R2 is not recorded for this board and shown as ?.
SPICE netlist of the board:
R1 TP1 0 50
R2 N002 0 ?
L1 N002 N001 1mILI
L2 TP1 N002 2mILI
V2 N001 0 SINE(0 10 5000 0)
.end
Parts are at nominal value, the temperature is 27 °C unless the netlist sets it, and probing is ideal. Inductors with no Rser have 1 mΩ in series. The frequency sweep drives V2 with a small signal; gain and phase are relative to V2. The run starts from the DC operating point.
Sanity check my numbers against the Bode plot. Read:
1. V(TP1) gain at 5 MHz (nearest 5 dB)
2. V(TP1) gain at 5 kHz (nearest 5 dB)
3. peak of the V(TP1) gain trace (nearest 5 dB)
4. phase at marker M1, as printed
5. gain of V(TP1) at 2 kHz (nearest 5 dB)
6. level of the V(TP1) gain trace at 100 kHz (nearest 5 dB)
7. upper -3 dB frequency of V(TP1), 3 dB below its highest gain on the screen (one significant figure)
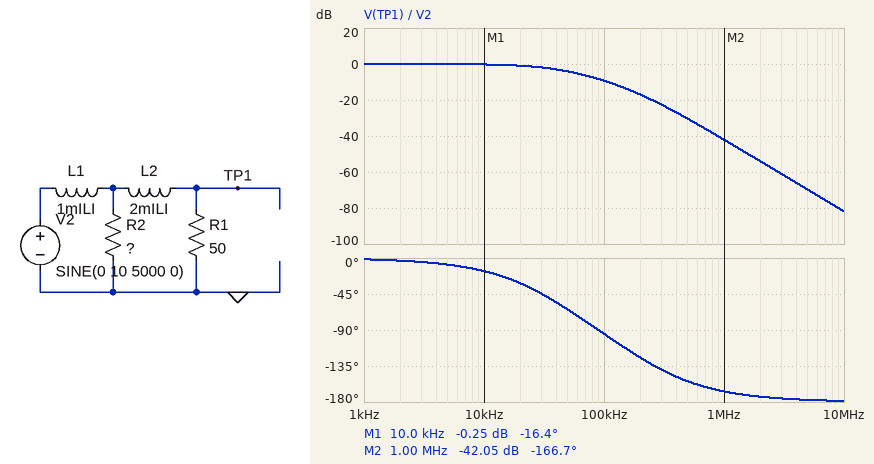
-70 dB
0 dB
0 dB
-16.4 deg
0 dB
-10 dB
40 kHz
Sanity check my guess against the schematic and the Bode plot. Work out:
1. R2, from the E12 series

8.2 Ω
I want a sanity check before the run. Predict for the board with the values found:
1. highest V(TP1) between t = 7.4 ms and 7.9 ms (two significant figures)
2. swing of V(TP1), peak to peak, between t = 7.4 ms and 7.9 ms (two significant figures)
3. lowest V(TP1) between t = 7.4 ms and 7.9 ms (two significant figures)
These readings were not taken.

9.9 V
20 V
-9.9 V
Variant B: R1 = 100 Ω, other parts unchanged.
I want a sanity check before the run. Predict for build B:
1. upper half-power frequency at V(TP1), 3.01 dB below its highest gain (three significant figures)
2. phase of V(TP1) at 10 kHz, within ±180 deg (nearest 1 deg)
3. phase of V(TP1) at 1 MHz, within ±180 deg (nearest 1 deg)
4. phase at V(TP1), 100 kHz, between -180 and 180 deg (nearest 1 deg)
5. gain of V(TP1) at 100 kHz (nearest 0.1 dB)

46.0 kHz
-14 deg
-158 deg
-81 deg
-7.8 dB
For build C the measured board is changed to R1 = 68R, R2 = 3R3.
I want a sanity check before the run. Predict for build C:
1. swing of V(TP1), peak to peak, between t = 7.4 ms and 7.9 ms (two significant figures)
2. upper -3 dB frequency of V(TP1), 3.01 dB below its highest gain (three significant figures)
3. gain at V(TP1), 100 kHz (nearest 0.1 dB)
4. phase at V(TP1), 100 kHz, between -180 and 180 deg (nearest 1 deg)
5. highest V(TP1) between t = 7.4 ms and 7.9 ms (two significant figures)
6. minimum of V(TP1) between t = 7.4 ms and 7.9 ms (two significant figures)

19 V
19.5 kHz
-15.1 dB
-103 deg
9.7 V
-9.7 V
